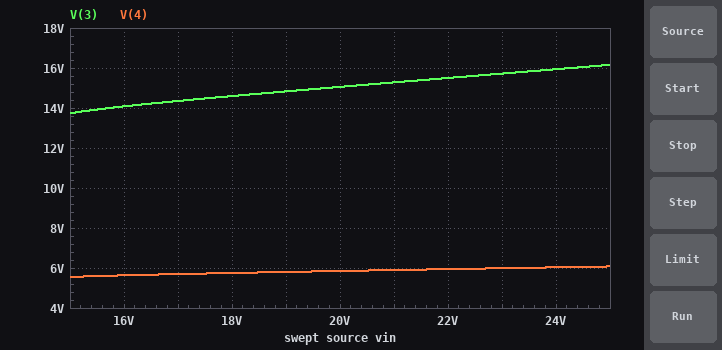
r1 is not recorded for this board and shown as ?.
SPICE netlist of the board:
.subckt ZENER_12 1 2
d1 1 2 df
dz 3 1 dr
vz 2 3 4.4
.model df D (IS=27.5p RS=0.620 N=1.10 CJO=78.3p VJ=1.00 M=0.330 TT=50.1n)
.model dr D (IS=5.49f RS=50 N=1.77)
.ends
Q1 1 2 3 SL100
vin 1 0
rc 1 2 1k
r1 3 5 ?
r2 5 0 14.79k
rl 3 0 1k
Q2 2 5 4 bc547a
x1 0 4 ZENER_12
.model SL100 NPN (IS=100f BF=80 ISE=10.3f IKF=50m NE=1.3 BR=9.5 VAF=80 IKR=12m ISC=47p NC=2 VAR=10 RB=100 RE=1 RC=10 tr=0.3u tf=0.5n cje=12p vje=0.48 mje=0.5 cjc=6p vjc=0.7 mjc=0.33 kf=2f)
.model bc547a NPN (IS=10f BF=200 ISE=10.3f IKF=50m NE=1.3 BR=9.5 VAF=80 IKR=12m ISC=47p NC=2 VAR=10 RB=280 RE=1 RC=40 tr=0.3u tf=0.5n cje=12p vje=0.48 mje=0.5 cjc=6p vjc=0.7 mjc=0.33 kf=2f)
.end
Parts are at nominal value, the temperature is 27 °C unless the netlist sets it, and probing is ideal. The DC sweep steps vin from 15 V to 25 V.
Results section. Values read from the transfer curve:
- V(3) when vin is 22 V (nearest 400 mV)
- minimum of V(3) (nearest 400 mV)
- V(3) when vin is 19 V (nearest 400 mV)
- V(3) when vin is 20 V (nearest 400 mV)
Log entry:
15.6 V
13.6 V
14.8 V
15.2 V
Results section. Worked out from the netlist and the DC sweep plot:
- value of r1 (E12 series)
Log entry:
18 kΩ
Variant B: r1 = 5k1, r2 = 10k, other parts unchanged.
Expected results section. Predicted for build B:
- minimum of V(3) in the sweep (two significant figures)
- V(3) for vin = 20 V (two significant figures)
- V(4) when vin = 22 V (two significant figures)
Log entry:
10 V
11 V
6.2 V
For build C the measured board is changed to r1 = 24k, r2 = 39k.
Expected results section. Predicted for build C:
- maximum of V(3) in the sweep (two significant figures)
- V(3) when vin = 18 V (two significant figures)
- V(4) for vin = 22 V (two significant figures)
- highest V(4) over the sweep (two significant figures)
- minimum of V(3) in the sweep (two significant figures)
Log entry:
13 V
12 V
6.1 V
6.2 V
11 V
